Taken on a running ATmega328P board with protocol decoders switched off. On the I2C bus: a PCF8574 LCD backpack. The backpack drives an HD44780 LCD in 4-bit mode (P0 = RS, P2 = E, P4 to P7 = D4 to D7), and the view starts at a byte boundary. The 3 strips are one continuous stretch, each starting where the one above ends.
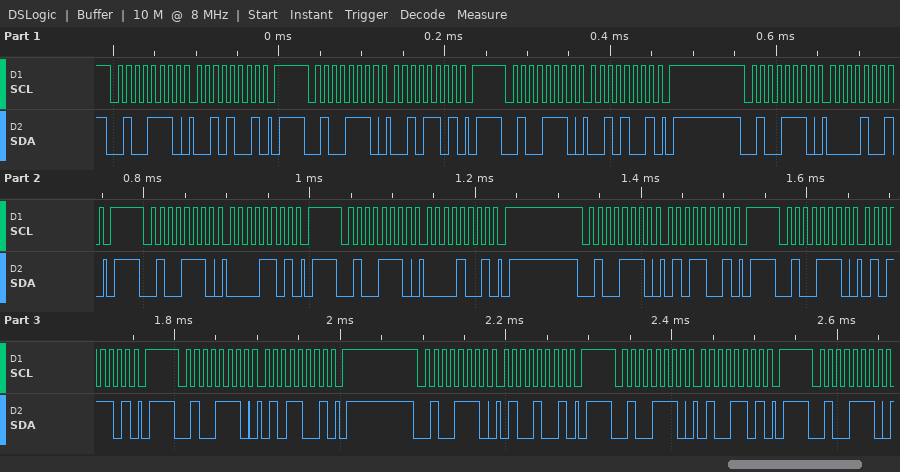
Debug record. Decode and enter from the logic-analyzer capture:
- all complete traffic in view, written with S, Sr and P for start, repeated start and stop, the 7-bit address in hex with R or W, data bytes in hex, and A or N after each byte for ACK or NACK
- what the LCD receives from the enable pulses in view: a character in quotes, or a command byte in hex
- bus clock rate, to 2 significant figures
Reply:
S 27W A 29 A P S 27W A 2D A P S 27W A 29 A P S 27W A 09 A P S 27W A 0D A P S 27W A 09 A P S 27W A 59 A P S 27W A 5D A P S 27W A 59 A P S 27W A 49 A P S 27W A 4D A P S 27W A
' '
100 kHz
